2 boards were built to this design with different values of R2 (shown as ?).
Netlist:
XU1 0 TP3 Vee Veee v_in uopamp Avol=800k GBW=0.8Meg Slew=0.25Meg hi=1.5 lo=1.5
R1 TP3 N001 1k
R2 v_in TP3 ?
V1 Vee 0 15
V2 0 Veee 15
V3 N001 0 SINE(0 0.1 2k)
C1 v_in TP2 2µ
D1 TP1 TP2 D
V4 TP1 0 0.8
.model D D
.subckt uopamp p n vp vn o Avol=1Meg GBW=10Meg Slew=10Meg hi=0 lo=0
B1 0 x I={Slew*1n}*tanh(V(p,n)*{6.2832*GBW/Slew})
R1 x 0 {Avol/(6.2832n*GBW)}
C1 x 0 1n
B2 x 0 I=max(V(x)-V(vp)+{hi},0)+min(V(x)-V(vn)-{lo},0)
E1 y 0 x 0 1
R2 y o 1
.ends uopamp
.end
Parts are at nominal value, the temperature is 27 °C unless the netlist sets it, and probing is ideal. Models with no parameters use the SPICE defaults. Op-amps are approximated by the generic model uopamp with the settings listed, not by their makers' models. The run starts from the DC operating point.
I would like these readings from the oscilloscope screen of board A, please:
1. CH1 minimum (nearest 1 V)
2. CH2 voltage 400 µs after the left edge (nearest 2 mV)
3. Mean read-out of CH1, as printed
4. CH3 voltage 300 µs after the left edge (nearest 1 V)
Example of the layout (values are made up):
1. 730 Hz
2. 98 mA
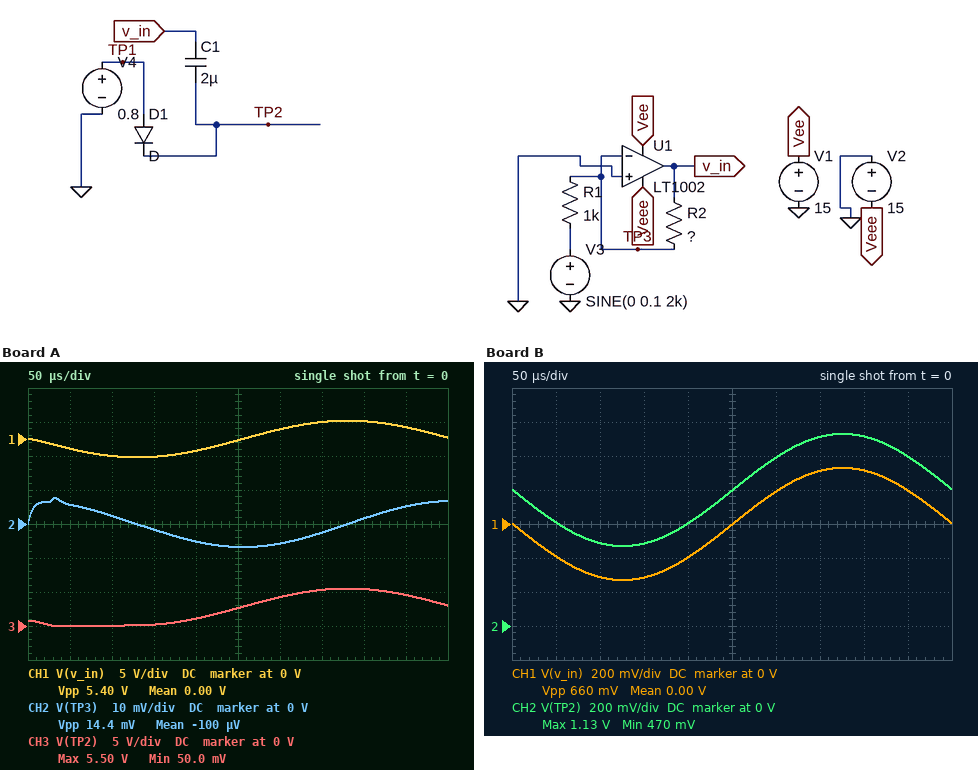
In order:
1. -3 V
2. 2 mV
3. 0.00 V
4. 4 V
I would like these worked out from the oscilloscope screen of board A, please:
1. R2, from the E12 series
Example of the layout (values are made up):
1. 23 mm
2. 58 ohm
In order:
1. 27 kΩ
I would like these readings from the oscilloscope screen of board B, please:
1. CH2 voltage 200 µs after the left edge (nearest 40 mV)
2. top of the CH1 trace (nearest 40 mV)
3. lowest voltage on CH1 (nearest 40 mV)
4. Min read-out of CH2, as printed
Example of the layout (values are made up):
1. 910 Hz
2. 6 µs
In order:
1. 600 mV
2. 320 mV
3. -320 mV
4. 470 mV
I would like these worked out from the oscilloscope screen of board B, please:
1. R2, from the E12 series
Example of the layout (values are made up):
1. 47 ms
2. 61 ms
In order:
1. 3.3 kΩ
